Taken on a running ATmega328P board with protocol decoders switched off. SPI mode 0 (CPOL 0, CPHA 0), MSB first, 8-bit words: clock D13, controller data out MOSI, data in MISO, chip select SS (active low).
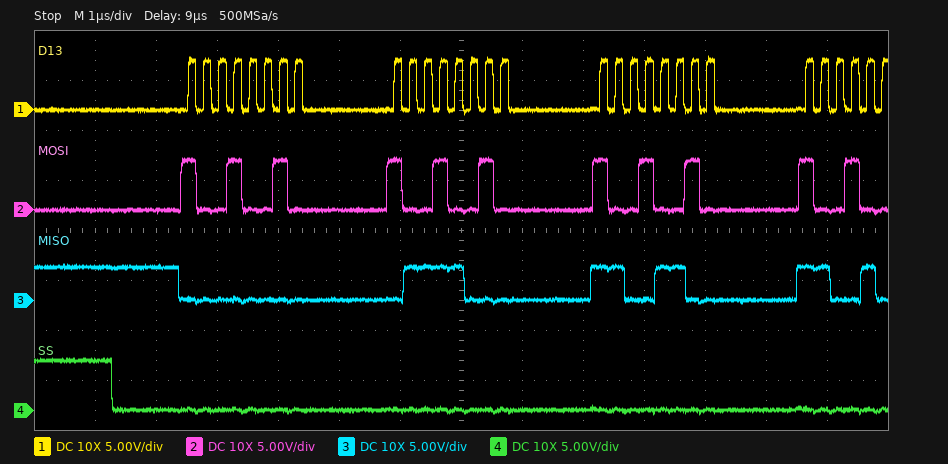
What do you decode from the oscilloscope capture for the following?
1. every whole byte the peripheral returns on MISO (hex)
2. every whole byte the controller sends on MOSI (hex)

00 78 CC
92 92 92
